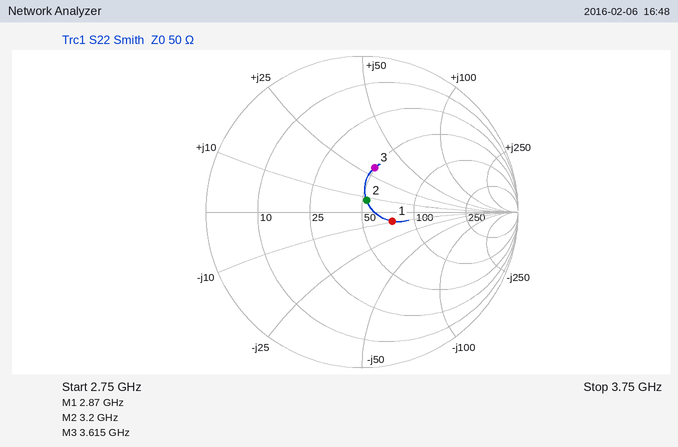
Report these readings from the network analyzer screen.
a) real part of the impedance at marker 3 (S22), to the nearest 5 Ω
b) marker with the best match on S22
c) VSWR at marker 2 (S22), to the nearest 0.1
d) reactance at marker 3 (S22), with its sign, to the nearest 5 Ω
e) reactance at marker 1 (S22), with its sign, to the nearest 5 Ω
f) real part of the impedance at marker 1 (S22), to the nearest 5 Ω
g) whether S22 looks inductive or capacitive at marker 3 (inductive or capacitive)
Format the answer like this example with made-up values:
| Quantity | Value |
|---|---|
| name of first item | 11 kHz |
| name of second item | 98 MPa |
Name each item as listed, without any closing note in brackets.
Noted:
| Quantity | Value |
|---|---|
| real part of the impedance at marker 3 (S22), to the nearest 5 Ω | 50 Ω |
| marker with the best match on S22 | marker 2 |
| VSWR at marker 2 (S22), to the nearest 0.1 | 1.2 |
| reactance at marker 3 (S22), with its sign, to the nearest 5 Ω | +30 Ω |
| reactance at marker 1 (S22), with its sign, to the nearest 5 Ω | -10 Ω |
| real part of the impedance at marker 1 (S22), to the nearest 5 Ω | 75 Ω |
| whether S22 looks inductive or capacitive at marker 3 | inductive |
